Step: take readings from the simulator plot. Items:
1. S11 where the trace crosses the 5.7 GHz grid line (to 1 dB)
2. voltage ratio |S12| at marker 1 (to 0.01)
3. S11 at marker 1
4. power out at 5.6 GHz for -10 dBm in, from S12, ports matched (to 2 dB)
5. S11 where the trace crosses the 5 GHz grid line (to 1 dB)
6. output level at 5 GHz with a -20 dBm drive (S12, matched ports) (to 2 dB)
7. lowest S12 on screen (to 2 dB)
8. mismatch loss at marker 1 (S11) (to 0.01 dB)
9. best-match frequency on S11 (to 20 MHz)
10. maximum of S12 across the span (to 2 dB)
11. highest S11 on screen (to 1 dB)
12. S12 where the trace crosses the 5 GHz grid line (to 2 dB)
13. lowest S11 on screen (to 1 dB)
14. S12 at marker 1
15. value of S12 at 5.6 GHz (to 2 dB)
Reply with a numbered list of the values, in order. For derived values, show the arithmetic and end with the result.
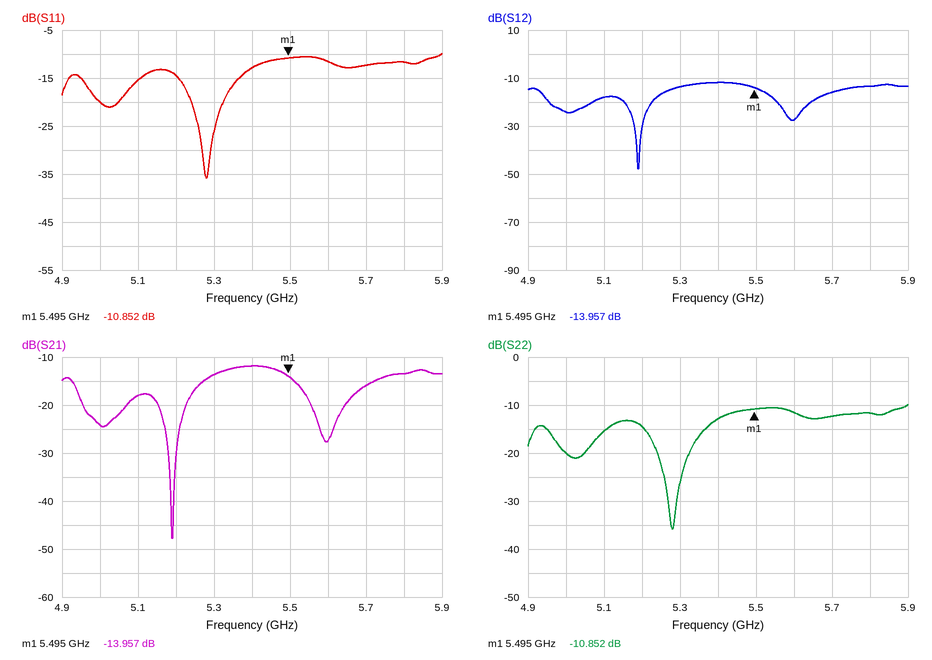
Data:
1. -12 dB
2. 10^(-13.957/20) ≈ 0.20
3. -10.852 dB
4. -10 dBm + (-28 dB) = -38 dBm
5. -20 dB
6. -20 dBm + (-24 dB) = -44 dBm
7. -48 dB
8. −10 log10(1 − 10^(-10.852/10)) ≈ 0.37 dB
9. 5.28 GHz
10. -12 dB
11. -10 dB
12. -24 dB
13. -36 dB
14. -13.957 dB
15. -28 dB
